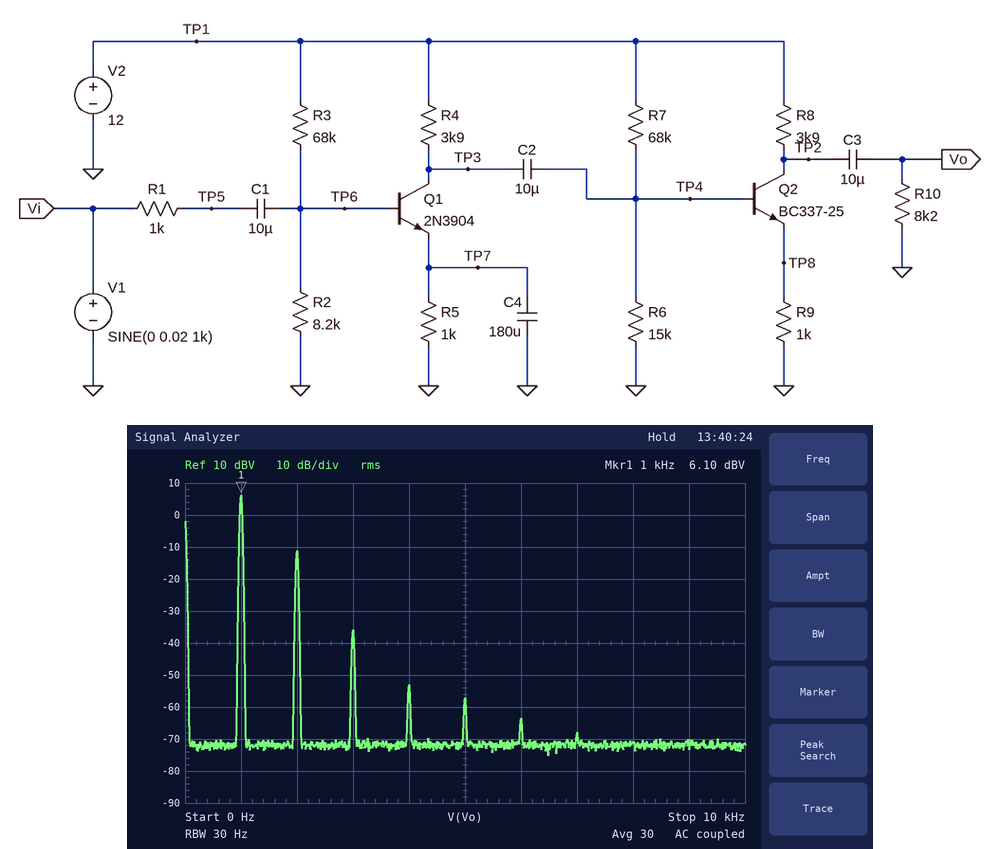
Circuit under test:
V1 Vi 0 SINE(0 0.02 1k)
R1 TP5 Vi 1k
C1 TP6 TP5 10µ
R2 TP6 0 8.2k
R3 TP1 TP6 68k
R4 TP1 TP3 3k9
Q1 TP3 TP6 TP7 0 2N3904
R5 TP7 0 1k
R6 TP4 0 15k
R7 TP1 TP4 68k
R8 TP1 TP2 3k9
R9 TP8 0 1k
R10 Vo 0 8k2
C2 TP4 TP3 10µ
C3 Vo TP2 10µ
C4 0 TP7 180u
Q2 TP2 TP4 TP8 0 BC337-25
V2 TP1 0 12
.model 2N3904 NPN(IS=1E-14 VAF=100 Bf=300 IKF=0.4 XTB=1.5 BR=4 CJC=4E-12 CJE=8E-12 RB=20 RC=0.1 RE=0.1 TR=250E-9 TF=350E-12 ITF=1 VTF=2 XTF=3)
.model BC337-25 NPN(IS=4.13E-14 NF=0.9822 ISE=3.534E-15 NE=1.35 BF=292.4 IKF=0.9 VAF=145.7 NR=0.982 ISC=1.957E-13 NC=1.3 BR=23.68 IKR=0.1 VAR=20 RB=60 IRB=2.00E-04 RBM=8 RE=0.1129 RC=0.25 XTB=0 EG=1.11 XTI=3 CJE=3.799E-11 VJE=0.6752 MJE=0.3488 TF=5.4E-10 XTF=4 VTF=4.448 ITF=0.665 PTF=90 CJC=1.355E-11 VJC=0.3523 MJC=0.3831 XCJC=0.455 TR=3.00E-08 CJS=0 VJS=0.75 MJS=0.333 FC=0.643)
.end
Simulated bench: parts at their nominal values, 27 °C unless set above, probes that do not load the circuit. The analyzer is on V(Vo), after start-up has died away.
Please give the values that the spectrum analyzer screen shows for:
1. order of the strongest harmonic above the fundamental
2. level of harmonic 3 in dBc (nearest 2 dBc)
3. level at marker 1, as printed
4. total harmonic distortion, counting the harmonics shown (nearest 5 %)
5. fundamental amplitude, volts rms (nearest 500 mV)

2
-42 dBc
6.10 dBV
15 %
2.0 V
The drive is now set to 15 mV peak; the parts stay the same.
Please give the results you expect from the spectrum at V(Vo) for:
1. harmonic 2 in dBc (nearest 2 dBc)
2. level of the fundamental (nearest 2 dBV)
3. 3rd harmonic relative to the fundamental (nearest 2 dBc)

-20 dBc
4 dBV
-46 dBc
